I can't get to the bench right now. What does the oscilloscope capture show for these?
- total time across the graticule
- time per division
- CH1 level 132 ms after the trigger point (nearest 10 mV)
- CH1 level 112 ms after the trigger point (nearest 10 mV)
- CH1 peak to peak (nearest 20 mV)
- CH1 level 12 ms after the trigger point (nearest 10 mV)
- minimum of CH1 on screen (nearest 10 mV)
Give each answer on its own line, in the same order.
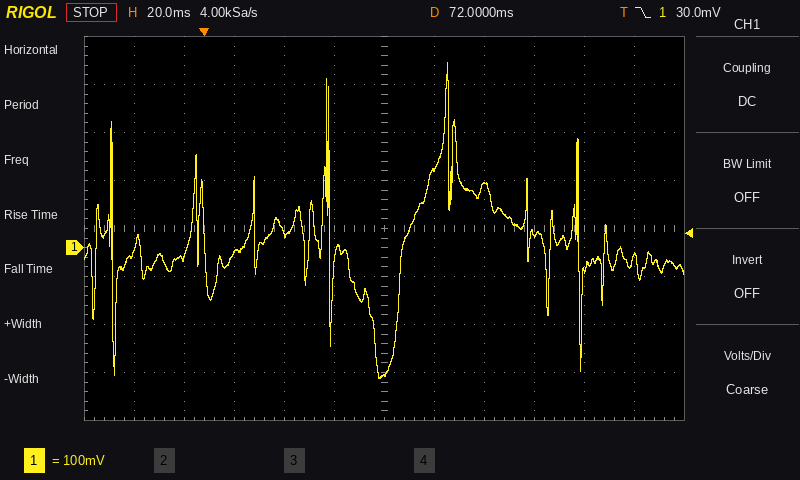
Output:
240 ms
20 ms
30 mV
130 mV
660 mV
-10 mV
-270 mV
